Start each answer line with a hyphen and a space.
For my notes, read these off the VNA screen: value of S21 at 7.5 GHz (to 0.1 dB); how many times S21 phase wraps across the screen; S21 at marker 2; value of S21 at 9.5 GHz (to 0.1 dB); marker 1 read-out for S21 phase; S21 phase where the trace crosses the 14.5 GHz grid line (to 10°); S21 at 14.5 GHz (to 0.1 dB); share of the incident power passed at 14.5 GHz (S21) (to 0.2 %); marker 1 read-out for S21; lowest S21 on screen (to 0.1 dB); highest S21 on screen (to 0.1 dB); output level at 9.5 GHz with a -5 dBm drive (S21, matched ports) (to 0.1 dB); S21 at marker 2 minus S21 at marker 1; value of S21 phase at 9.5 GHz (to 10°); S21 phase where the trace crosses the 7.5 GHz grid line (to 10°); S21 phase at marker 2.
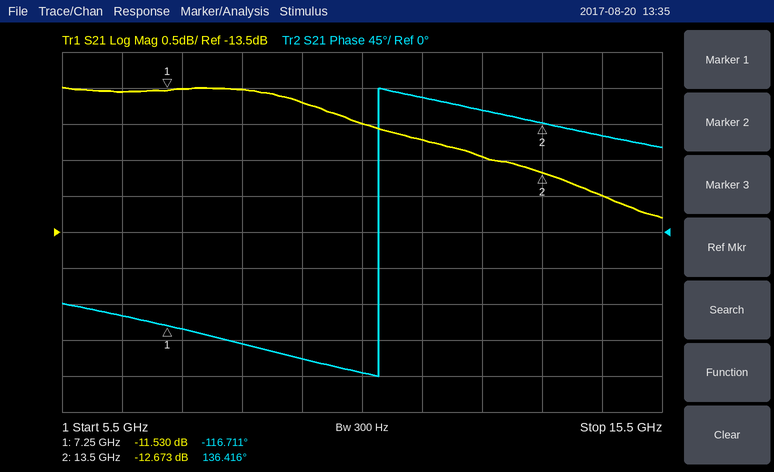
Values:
- -11.5 dB
- 1
- -12.673 dB
- -11.7 dB
- -116.711°
- 120°
- -13.0 dB
- 5.0 %
- -11.530 dB
- -13.3 dB
- -11.5 dB
- -16.7 dBm
- -1.143 dB
- -160°
- -120°
- 136.416°
